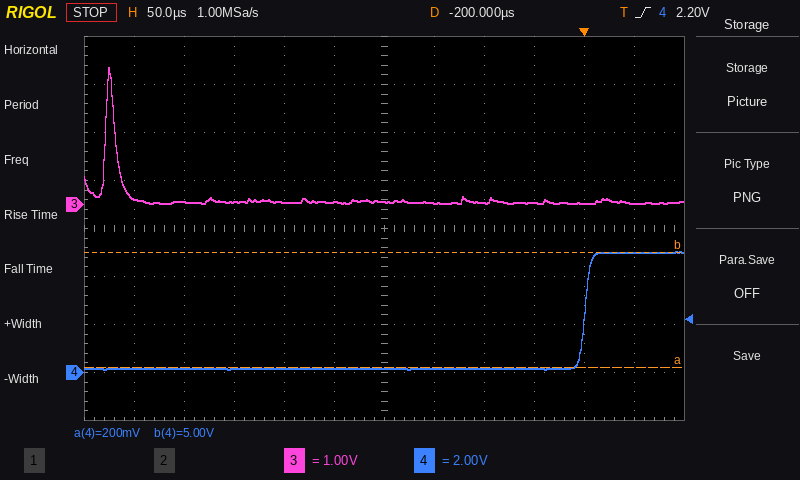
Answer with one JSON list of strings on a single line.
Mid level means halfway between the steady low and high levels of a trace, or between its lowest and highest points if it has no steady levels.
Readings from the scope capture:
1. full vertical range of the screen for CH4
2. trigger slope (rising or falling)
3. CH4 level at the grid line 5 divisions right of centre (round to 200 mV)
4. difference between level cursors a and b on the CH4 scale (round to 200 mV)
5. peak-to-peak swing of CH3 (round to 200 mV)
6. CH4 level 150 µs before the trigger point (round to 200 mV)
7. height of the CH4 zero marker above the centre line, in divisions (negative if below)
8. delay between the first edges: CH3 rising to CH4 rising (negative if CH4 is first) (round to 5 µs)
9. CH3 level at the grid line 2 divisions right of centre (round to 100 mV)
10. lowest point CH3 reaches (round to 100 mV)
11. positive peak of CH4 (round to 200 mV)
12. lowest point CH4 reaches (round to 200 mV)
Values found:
["16 V", "rising", "5.0 V", "4.8 V", "2.8 V", "200 mV", "-3.0 div", "+480 µs", "0.0 V", "0.0 V", "5.0 V", "200 mV"]
